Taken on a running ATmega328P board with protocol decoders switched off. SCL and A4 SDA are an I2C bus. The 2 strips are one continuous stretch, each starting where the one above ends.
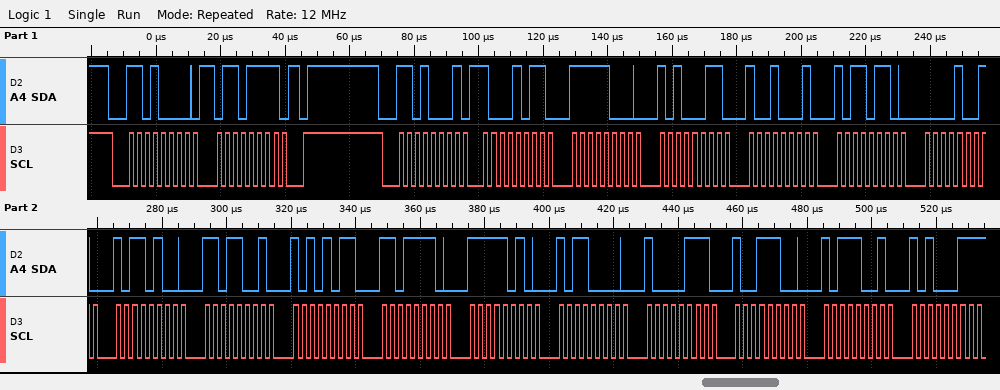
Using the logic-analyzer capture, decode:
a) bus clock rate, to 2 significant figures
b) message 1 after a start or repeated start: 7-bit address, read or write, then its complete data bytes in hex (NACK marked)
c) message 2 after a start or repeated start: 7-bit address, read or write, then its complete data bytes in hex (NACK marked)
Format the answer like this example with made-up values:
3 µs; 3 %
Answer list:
400 kHz; 0x68 write: 6F; 0x68 read: 8B F8 A3 91 B6 09 B4 D9 AB DE FA B0 87 9C B9 A3 NACK
